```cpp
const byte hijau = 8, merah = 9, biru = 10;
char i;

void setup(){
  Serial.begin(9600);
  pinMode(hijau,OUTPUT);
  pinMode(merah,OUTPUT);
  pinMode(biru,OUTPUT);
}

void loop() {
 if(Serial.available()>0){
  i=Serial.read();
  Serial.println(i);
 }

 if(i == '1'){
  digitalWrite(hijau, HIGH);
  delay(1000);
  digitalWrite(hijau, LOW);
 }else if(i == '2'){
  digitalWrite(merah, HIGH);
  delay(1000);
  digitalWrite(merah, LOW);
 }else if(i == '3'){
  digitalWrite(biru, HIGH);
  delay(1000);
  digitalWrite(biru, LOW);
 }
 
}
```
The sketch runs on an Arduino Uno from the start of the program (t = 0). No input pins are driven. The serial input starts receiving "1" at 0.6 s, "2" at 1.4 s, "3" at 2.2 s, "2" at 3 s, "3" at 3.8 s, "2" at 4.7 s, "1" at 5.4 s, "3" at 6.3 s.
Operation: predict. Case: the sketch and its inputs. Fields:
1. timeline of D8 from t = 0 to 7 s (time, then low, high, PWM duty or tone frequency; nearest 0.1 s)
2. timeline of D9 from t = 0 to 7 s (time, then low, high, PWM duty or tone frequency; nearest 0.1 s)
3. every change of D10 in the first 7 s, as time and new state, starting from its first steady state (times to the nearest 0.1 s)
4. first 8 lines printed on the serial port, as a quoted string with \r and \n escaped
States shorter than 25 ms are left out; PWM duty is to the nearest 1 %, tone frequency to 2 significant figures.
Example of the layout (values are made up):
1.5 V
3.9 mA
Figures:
0 s low; 0.6 s high; 1.6 s low; 6.6 s high
0 s low; 1.6 s high; 2.6 s low; 3.6 s high; 4.6 s low; 5.6 s high; 6.6 s low
0 s low; 2.6 s high; 3.6 s low; 4.6 s high; 5.6 s low
"1\r\n2\r\n3\r\n2\r\n3\r\n2\r\n1\r\n3\r\n"
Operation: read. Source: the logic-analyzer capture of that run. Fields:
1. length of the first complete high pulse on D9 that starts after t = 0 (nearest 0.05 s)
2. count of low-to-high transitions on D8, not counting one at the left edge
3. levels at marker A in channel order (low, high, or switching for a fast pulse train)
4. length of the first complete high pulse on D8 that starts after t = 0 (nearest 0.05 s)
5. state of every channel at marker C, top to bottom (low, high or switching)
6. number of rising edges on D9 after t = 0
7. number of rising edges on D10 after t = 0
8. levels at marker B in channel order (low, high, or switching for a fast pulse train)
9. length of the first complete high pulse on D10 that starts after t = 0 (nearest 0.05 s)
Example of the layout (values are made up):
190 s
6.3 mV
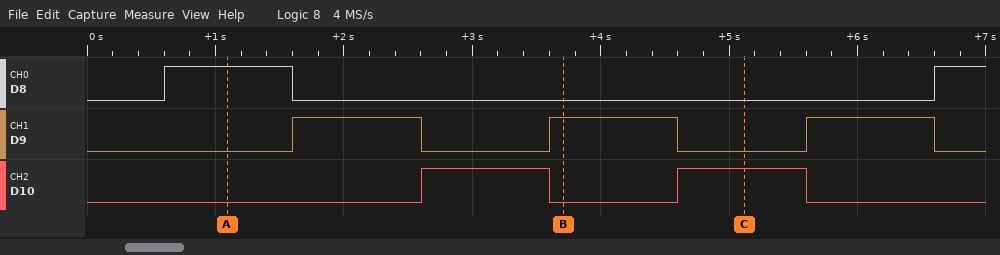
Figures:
1.00 s
2
D8 high, D9 low, D10 low
1.00 s
D8 low, D9 low, D10 high
3
2
D8 low, D9 high, D10 low
1.00 s
